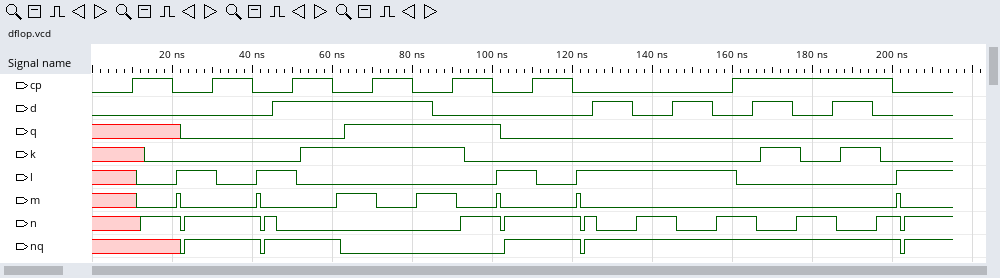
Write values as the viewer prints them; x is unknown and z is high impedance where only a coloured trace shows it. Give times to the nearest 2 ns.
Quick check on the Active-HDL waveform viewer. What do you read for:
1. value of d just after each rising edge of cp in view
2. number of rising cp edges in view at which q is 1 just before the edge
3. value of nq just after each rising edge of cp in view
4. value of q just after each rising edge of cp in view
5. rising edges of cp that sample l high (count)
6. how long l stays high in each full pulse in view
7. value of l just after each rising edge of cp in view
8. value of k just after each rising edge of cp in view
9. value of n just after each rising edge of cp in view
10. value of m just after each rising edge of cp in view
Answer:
0 0 1 1 0 0 0
2
x 1 1 0 0 1 1
x 0 0 1 1 0 0
4
10 ns, 10 ns, 10 ns, 40 ns
x 1 1 0 0 1 1
x 0 0 1 1 0 0
x 1 0 0 0 1 1
x 0 0 1 1 0 0
